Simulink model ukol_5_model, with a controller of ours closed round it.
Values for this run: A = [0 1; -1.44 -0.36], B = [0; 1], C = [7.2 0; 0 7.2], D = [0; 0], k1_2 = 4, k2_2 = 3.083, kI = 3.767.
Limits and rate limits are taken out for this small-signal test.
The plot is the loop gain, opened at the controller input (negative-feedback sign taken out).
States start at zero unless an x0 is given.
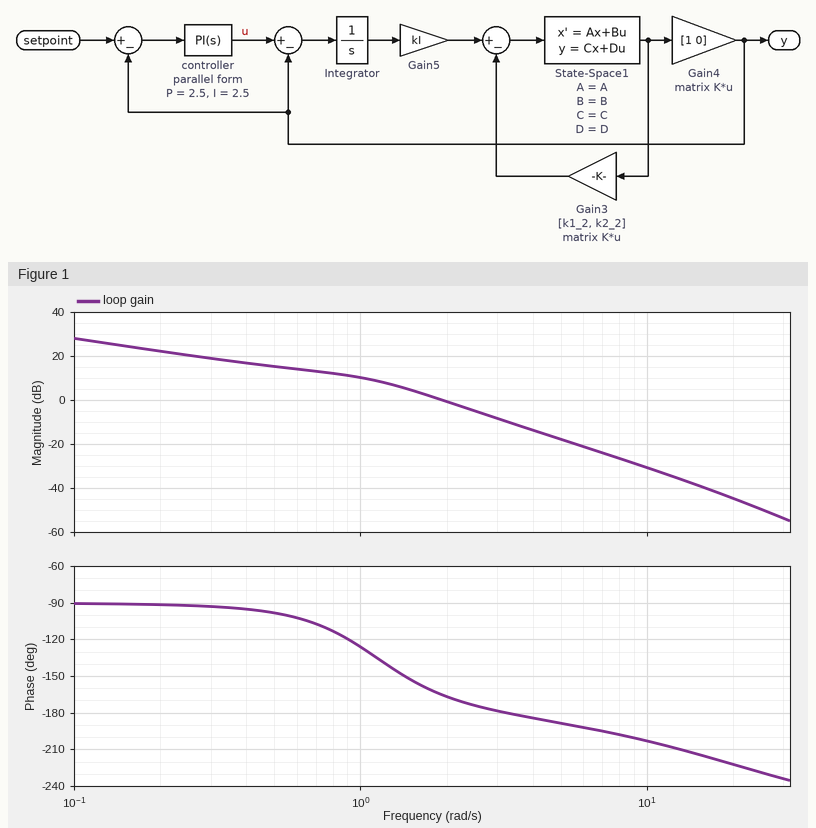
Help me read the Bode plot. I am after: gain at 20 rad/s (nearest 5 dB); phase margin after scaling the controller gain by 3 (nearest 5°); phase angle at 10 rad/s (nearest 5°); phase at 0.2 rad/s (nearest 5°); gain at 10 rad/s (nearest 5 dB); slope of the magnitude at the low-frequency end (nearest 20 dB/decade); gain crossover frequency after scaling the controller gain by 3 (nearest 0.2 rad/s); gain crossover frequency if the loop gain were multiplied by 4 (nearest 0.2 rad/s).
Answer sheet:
-45 dB
0°
-205°
-90°
-30 dB
-20 dB/decade
3.2 rad/s
3.6 rad/s
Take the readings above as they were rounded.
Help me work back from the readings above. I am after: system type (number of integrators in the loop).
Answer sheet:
1
